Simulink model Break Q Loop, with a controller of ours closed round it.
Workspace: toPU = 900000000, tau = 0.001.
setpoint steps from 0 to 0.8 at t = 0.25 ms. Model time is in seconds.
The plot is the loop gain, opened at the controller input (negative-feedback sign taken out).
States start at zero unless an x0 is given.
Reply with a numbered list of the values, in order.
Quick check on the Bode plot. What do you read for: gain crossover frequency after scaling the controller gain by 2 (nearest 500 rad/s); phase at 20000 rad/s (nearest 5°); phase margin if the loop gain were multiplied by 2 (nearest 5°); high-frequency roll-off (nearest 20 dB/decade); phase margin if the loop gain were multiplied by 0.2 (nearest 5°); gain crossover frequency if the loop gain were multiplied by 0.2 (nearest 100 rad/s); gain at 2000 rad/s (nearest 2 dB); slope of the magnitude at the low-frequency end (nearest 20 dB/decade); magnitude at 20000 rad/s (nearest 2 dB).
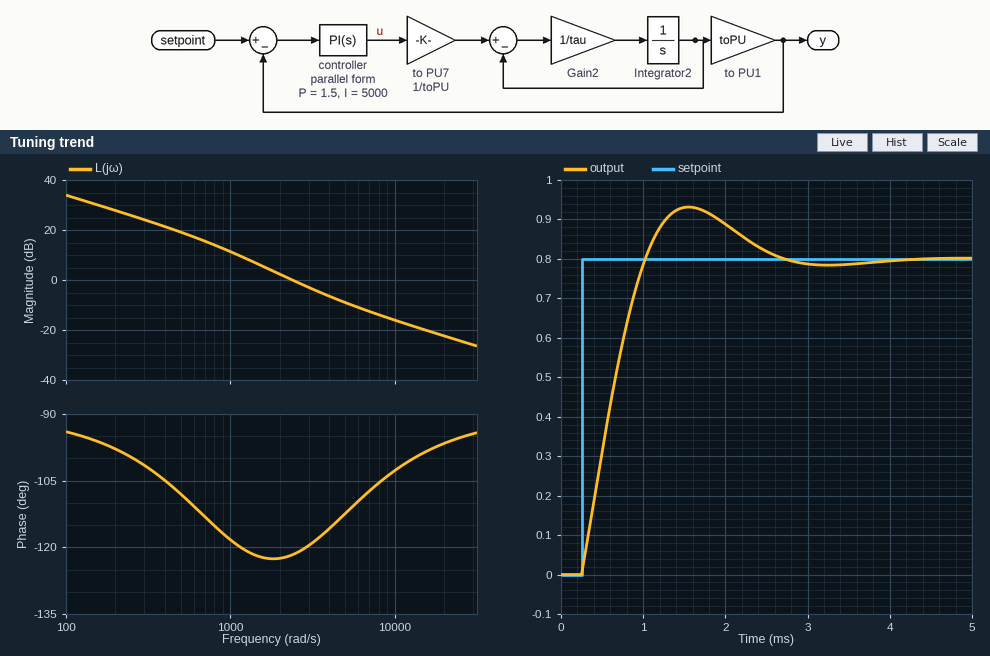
1. 4000 rad/s
2. -95°
3. 65°
4. -20 dB/decade
5. 65°
6. 800 rad/s
7. 2 dB
8. -20 dB/decade
9. -22 dB
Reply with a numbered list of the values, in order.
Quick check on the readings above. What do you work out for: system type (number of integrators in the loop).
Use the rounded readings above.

1. 1
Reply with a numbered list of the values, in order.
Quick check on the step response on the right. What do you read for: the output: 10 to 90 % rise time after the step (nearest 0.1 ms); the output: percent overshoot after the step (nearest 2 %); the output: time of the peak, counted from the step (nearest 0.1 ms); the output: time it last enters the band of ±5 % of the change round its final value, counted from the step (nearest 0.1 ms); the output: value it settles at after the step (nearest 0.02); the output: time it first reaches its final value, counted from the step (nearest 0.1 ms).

1. 0.6 ms
2. 16 %
3. 1.3 ms
4. 2.1 ms
5. 0.80
6. 0.8 ms
